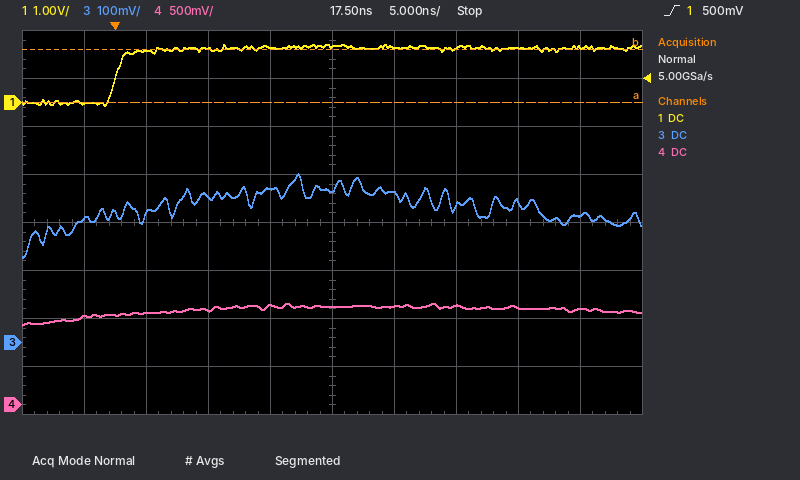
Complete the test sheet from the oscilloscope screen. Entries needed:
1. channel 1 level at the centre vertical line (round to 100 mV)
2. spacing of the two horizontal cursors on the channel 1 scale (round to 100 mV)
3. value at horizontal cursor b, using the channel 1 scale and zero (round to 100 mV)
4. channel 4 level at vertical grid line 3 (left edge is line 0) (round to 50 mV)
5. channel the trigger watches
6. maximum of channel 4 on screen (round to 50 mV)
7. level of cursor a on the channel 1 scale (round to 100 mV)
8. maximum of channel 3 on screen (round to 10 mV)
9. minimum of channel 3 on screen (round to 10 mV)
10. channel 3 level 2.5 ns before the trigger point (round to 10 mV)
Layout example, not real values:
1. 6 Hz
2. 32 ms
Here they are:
1. 1.2 V
2. 1.1 V
3. 1.1 V
4. 1.00 V
5. channel 1
6. 1.05 V
7. 0.0 V
8. 350 mV
9. 180 mV
10. 260 mV
